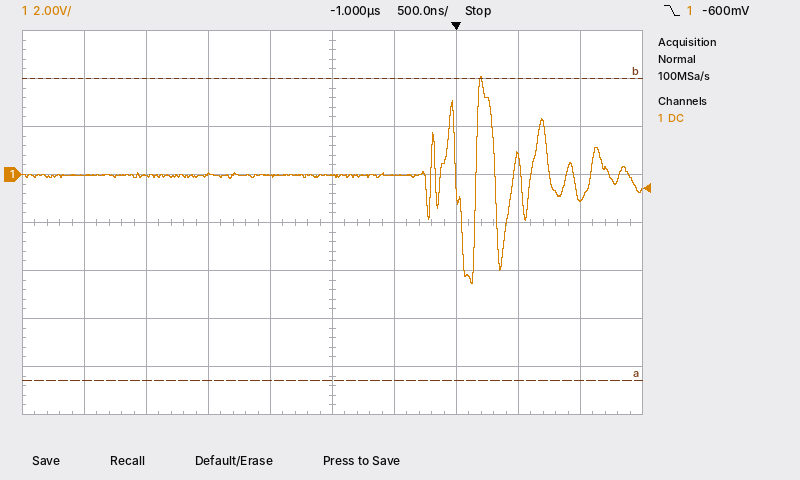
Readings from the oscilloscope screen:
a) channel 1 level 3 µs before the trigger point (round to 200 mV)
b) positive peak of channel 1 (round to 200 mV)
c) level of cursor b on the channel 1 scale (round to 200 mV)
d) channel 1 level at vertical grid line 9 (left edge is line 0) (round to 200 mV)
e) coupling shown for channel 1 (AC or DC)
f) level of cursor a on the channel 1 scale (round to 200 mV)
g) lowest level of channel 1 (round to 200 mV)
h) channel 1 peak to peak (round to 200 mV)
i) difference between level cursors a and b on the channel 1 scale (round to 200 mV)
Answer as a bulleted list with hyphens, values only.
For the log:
- 0.0 V
- 4.0 V
- 4.0 V
- -1.0 V
- DC
- -8.6 V
- -4.6 V
- 8.6 V
- 12.6 V
